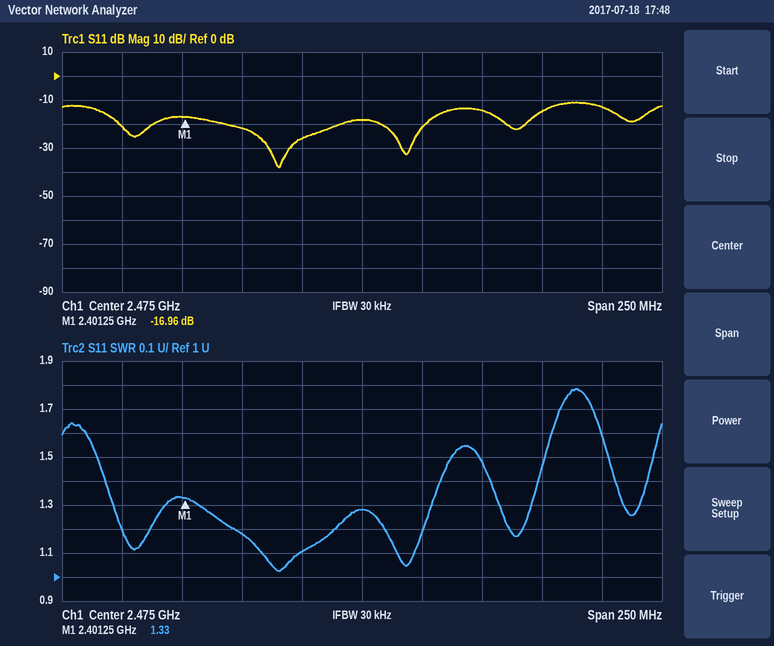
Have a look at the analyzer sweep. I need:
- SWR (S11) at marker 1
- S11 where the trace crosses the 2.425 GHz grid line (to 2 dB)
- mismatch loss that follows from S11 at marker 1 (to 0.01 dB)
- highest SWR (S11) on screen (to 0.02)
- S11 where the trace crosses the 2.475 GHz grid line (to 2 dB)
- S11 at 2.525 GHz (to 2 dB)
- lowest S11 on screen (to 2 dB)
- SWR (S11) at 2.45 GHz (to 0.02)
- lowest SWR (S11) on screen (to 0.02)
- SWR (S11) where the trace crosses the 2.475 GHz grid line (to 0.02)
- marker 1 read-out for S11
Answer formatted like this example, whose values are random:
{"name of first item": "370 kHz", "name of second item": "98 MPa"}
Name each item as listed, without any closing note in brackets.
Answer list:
{"SWR (S11) at marker 1": "1.33", "S11 where the trace crosses the 2.425 GHz grid line": "-22 dB", "mismatch loss that follows from S11 at marker 1": "0.09 dB", "highest SWR (S11) on screen": "1.78", "S11 where the trace crosses the 2.475 GHz grid line": "-18 dB", "S11 at 2.525 GHz": "-14 dB", "lowest S11 on screen": "-38 dB", "SWR (S11) at 2.45 GHz": "1.10", "lowest SWR (S11) on screen": "1.02", "SWR (S11) where the trace crosses the 2.475 GHz grid line": "1.28", "marker 1 read-out for S11": "-16.96 dB"}
